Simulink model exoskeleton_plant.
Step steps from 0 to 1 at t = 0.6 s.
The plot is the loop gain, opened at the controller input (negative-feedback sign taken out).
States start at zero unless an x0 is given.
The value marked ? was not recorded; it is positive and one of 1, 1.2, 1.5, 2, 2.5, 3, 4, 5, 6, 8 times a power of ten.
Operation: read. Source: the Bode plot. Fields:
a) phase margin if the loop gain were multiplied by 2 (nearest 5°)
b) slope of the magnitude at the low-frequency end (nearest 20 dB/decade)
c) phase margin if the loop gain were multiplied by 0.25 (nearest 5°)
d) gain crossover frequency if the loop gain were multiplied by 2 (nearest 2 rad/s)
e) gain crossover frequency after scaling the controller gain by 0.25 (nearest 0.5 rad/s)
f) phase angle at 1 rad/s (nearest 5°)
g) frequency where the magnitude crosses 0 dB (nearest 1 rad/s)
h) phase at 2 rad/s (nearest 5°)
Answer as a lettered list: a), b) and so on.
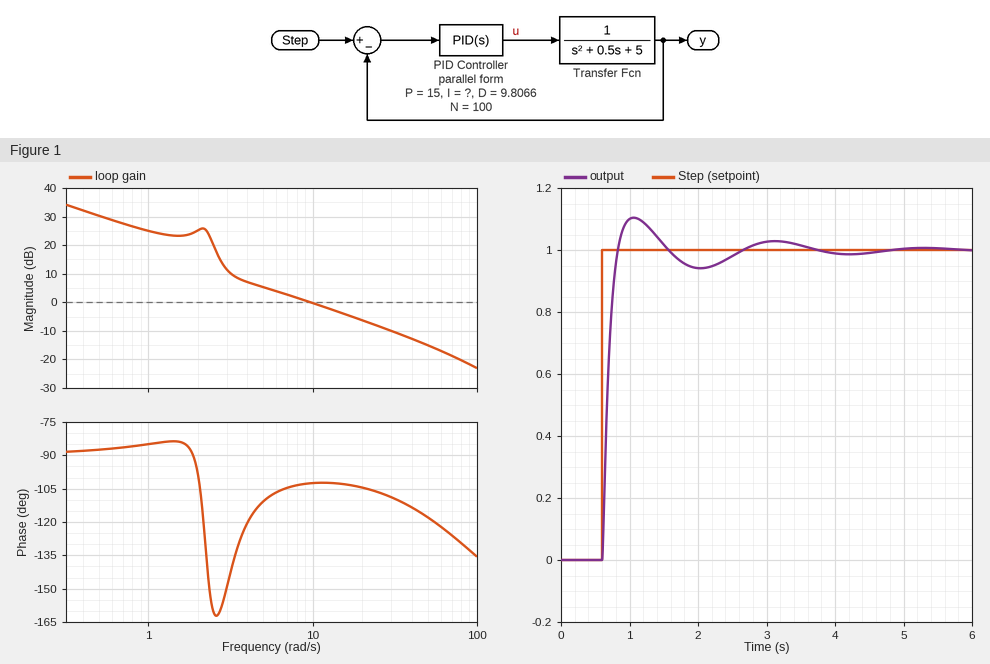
a) 75°
b) -20 dB/decade
c) 30°
d) 20 rad/s
e) 3.0 rad/s
f) -85°
g) 10 rad/s
h) -100°
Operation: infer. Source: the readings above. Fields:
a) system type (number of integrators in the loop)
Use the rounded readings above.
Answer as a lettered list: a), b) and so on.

a) 1
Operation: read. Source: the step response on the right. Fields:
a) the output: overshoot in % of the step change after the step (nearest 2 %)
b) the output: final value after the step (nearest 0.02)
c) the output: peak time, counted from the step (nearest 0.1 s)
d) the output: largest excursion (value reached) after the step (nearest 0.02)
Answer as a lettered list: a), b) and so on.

a) 10 %
b) 1.00
c) 0.5 s
d) 1.10
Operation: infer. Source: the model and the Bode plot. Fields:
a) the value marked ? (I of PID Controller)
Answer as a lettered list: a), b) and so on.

a) 80
